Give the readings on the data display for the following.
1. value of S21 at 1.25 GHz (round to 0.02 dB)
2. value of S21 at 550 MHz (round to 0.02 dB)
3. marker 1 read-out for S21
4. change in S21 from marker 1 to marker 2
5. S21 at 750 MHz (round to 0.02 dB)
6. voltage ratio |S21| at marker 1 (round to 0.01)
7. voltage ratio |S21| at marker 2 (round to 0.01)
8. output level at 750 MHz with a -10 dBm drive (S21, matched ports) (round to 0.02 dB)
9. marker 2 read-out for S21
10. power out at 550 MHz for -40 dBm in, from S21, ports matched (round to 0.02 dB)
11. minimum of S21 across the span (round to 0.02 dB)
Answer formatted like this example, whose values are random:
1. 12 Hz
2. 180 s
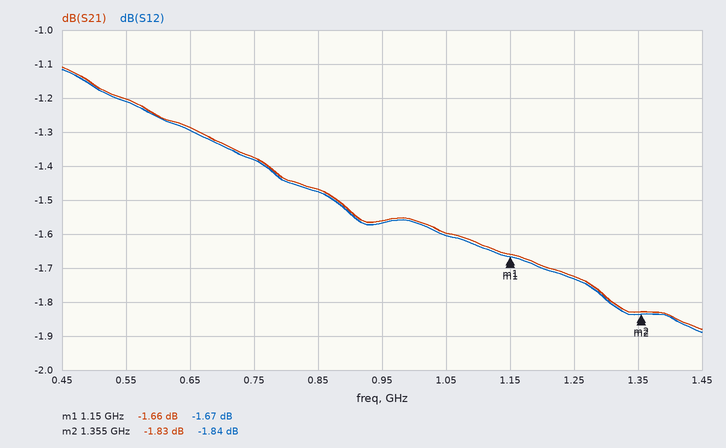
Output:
1. -1.72 dB
2. -1.20 dB
3. -1.66 dB
4. -0.17 dB
5. -1.38 dB
6. 0.83
7. 0.81
8. -11.38 dBm
9. -1.83 dB
10. -41.20 dBm
11. -1.88 dB
